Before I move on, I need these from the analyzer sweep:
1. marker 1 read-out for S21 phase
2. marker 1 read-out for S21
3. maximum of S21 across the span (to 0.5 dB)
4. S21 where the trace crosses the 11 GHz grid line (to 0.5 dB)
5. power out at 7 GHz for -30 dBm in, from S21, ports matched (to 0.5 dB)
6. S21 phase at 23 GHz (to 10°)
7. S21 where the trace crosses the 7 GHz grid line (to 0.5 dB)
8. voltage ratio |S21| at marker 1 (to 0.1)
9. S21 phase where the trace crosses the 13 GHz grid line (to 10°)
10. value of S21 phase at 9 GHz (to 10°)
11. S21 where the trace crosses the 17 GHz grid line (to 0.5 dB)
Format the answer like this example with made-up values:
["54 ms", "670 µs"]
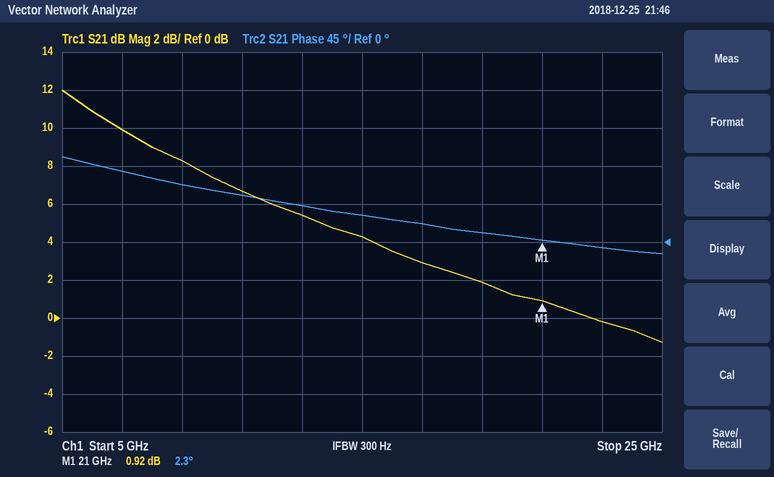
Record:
["2.3°", "0.92 dB", "12.0 dB", "6.5 dB", "-20.0 dBm", "-10°", "10.0 dB", "1.1", "40°", "70°", "3.0 dB"]
